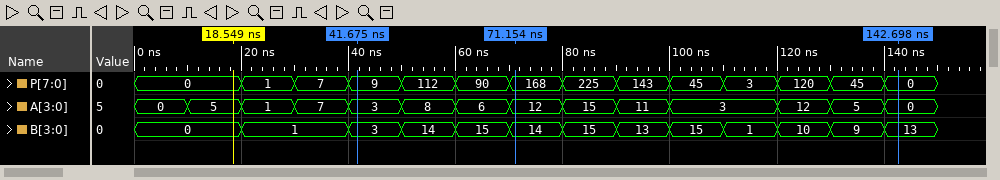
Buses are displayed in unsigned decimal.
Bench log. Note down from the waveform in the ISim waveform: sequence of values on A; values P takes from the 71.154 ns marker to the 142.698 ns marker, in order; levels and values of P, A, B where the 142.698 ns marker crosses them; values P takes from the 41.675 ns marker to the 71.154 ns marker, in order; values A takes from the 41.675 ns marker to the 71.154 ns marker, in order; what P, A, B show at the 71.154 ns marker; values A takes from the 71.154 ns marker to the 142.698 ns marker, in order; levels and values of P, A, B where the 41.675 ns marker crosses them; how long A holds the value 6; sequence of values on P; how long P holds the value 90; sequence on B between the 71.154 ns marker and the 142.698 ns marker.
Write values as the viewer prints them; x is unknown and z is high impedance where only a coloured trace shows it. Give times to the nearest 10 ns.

0, 5, 1, 7, 3, 8, 6, 12, 15, 11, 3, 12, 5, 0
168, 225, 143, 45, 3, 120, 45, 0
P=0, A=0, B=13
9, 112, 90, 168
3, 8, 6, 12
P=168, A=12, B=14
12, 15, 11, 3, 12, 5, 0
P=9, A=3, B=3
10 ns
0, 1, 7, 9, 112, 90, 168, 225, 143, 45, 3, 120, 45, 0
10 ns
14, 15, 13, 15, 1, 10, 9, 13
